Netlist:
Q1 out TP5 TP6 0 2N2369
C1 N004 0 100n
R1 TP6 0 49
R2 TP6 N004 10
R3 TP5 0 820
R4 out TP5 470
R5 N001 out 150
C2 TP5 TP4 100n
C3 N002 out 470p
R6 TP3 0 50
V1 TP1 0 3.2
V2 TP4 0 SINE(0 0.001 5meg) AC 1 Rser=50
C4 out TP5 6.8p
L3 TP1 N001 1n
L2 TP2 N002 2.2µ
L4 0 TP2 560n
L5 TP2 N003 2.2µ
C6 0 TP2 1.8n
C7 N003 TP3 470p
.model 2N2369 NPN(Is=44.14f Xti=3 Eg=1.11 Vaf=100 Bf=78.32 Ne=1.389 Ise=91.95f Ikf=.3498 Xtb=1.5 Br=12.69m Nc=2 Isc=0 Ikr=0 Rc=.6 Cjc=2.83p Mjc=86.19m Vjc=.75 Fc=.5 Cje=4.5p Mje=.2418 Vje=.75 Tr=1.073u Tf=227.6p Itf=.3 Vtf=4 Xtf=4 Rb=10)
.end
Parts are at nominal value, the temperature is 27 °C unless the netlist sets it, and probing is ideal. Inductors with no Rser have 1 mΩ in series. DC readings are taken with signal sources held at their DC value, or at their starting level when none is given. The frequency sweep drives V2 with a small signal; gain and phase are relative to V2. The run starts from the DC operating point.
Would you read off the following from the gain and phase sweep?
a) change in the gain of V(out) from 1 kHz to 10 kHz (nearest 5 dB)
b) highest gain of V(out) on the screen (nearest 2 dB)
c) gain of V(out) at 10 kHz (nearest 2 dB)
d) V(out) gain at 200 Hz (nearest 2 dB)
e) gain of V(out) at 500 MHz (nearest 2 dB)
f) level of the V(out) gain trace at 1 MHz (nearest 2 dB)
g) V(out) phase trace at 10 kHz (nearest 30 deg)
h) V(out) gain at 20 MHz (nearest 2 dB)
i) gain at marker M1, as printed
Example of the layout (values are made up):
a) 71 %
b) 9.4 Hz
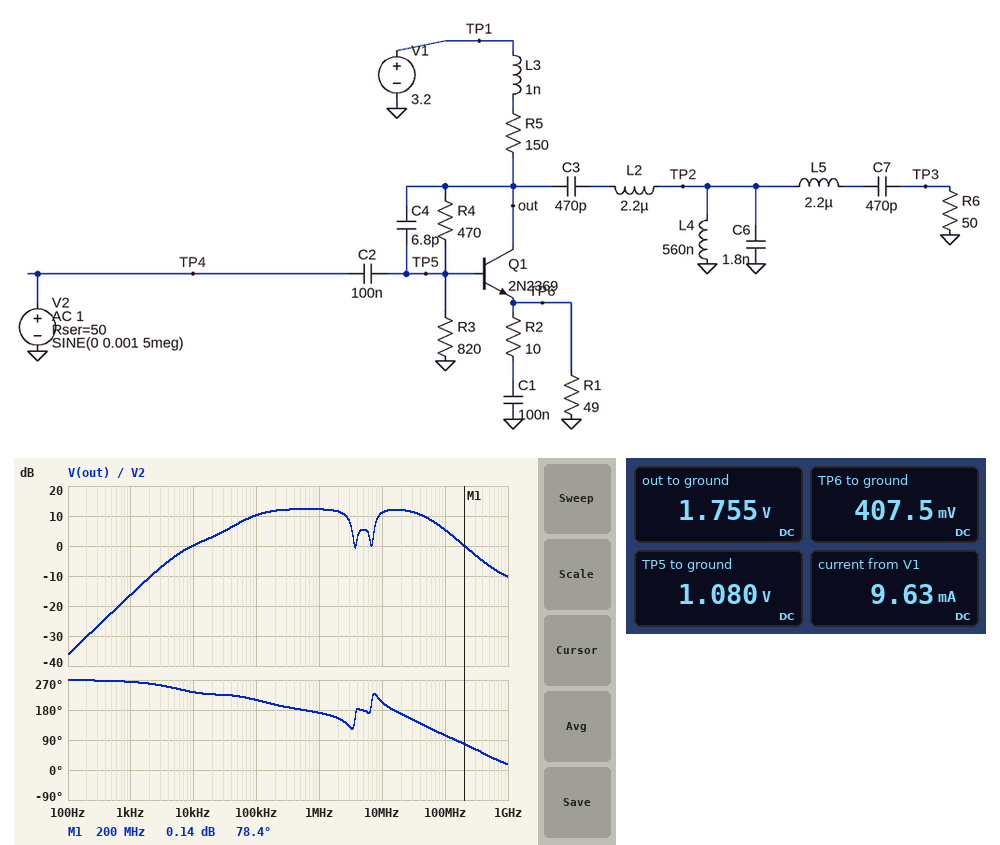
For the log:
a) 15 dB
b) 12 dB
c) 0 dB
d) -30 dB
e) -6 dB
f) 12 dB
g) 240 deg
h) 12 dB
i) 0.14 dB
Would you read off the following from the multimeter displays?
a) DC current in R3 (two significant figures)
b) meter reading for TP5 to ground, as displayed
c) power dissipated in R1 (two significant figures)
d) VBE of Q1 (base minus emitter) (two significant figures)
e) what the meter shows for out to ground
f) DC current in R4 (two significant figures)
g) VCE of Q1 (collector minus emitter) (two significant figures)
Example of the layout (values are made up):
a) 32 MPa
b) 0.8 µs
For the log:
a) 1.3 mA
b) 1.080 V
c) 3.4 mW
d) 670 mV
e) 1.755 V
f) 1.4 mA
g) 1.3 V
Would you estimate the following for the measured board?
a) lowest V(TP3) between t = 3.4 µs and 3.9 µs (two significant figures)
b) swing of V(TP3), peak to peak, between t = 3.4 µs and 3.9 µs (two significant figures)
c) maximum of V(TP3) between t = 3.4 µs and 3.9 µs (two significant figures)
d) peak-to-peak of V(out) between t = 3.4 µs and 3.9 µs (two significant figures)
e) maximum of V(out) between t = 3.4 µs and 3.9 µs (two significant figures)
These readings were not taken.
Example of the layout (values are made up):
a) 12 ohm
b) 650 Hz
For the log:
a) -1.9 mV
b) 3.7 mV
c) 1.9 mV
d) 3.7 mV
e) 1.8 V
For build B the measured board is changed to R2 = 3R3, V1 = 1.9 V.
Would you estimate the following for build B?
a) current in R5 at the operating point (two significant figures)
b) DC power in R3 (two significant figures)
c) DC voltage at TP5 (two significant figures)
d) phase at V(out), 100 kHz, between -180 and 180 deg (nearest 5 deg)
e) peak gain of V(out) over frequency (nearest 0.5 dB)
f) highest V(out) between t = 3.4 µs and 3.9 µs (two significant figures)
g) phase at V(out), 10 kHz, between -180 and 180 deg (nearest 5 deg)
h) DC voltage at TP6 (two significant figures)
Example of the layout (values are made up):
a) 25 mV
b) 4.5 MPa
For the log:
a) 4.1 mA
b) 780 µW
c) 800 mV
d) -145 deg
e) 12.5 dB
f) 1.3 V
g) -130 deg
h) 150 mV
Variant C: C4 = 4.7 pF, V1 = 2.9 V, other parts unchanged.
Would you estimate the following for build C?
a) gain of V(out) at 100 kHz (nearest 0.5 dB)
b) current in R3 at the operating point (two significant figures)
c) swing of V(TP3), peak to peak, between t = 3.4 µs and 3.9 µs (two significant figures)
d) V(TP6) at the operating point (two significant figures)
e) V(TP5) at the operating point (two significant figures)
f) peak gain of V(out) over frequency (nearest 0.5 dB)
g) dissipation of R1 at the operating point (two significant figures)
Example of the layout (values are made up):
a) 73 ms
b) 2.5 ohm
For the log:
a) 10.0 dB
b) 1.2 mA
c) 3.6 mV
d) 350 mV
e) 1.0 V
f) 12.0 dB
g) 2.5 mW
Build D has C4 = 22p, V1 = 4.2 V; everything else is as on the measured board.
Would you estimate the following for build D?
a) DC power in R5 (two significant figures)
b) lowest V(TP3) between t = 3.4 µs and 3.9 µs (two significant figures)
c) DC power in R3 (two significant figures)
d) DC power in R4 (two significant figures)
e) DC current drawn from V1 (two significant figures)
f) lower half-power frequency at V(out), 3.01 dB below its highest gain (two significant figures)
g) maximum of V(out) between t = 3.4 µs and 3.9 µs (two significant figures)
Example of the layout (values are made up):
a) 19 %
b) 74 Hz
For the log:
a) 29 mW
b) -2.0 mV
c) 2.0 mW
d) 1.4 mW
e) 14 mA
f) 78 kHz
g) 2.1 V
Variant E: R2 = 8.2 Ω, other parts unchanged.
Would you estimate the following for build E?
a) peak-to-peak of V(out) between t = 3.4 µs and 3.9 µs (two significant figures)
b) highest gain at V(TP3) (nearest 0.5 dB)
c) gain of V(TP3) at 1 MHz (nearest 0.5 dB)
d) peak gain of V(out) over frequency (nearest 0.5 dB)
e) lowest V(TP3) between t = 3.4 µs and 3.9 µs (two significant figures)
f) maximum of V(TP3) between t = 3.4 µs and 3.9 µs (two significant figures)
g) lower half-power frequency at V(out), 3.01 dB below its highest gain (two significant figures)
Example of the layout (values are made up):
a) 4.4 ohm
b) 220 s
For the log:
a) 4.1 mV
b) 6.0 dB
c) -42.5 dB
d) 13.0 dB
e) -2.0 mV
f) 2.0 mV
g) 83 kHz
